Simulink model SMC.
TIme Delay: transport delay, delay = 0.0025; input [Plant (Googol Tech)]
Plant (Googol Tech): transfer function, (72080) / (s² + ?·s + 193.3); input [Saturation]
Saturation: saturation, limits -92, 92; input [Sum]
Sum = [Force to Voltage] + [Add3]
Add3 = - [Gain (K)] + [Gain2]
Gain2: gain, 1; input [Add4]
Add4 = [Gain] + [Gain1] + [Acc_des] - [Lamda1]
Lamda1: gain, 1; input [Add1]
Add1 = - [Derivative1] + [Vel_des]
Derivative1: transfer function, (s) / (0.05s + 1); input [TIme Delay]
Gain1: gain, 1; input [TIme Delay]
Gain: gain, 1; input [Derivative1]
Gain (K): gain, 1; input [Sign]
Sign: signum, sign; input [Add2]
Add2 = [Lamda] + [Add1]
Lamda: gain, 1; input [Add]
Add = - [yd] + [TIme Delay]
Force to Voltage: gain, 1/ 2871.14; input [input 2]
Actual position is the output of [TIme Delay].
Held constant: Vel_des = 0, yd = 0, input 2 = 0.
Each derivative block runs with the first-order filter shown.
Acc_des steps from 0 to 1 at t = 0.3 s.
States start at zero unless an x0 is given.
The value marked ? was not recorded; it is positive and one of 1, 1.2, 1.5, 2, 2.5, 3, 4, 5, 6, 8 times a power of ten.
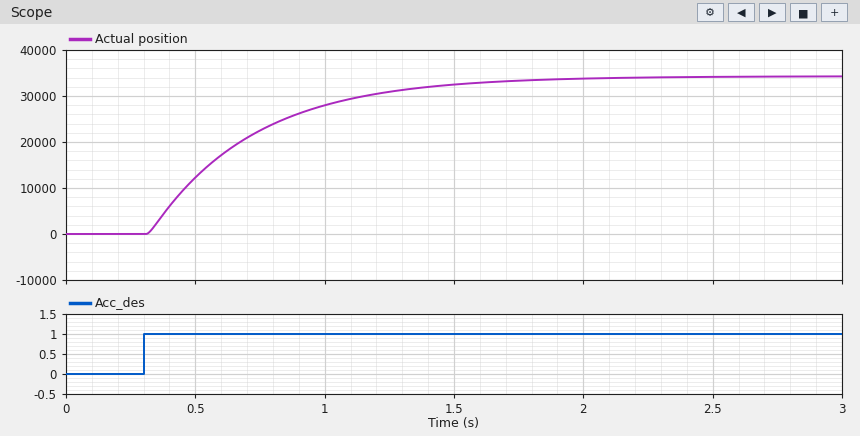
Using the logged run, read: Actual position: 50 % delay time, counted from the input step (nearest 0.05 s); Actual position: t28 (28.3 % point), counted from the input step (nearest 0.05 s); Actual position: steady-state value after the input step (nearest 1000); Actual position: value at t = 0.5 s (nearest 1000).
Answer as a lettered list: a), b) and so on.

a) 0.30 s
b) 0.15 s
c) 34000
d) 12000
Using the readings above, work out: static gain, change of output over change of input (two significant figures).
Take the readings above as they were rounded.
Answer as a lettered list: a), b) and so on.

a) 34000
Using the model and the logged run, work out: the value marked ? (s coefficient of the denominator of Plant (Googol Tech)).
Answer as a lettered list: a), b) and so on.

a) 80
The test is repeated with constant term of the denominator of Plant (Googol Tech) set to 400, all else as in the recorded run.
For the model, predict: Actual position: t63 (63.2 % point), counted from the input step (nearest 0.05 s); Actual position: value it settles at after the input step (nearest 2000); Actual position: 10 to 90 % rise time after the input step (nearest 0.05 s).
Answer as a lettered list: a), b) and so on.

a) 0.20 s
b) 16000
c) 0.40 s
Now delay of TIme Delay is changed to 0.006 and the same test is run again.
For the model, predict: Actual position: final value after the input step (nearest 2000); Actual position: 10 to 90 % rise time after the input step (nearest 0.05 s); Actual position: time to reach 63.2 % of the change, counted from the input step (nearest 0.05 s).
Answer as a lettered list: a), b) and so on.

a) 34000
b) 0.90 s
c) 0.45 s
